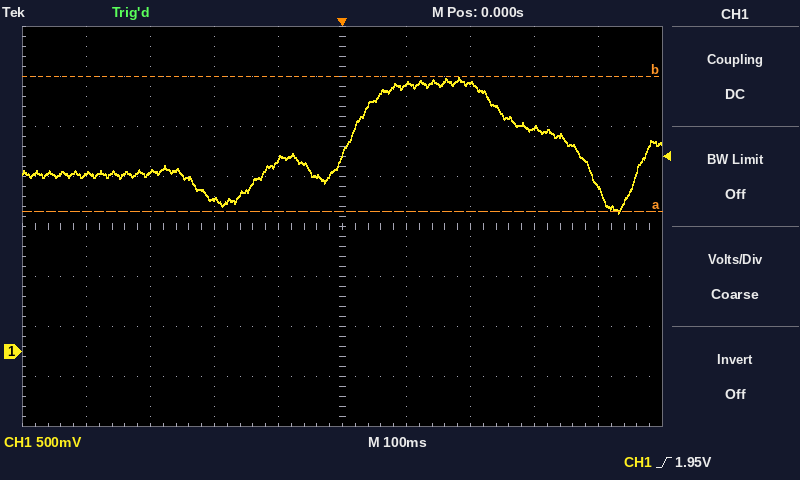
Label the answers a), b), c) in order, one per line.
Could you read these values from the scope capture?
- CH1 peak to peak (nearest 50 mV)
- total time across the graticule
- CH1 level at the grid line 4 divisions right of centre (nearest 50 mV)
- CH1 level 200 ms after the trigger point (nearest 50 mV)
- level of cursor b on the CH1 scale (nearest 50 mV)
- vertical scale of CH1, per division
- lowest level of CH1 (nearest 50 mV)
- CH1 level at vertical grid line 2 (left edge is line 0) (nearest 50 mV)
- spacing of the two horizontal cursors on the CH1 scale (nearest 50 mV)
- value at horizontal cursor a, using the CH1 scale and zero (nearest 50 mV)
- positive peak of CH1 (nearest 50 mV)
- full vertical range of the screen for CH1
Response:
a) 1.35 V
b) 1 s
c) 1.65 V
d) 2.70 V
e) 2.75 V
f) 500 mV
g) 1.40 V
h) 1.80 V
i) 1.35 V
j) 1.40 V
k) 2.75 V
l) 4 V
